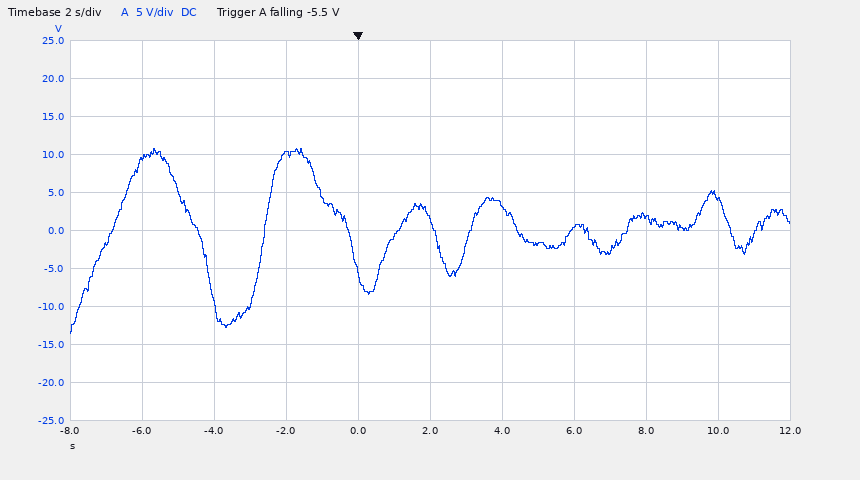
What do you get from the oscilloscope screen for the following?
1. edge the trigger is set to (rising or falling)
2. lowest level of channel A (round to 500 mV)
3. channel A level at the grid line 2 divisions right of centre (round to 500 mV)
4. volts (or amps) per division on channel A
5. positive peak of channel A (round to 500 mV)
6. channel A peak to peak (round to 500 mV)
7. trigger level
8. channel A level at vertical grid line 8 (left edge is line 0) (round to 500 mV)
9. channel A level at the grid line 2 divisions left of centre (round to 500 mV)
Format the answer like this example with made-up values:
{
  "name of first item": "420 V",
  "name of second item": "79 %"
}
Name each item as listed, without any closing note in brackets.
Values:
{
  "edge the trigger is set to": "falling",
  "lowest level of channel A": "-13.5 V",
  "channel A level at the grid line 2 divisions right of centre": "500 mV",
  "volts (or amps) per division on channel A": "5 V",
  "positive peak of channel A": "11.0 V",
  "channel A peak to peak": "24.5 V",
  "trigger level": "-5.5 V",
  "channel A level at vertical grid line 8 (left edge is line 0)": "2.0 V",
  "channel A level at the grid line 2 divisions left of centre": "10.0 V"
}
